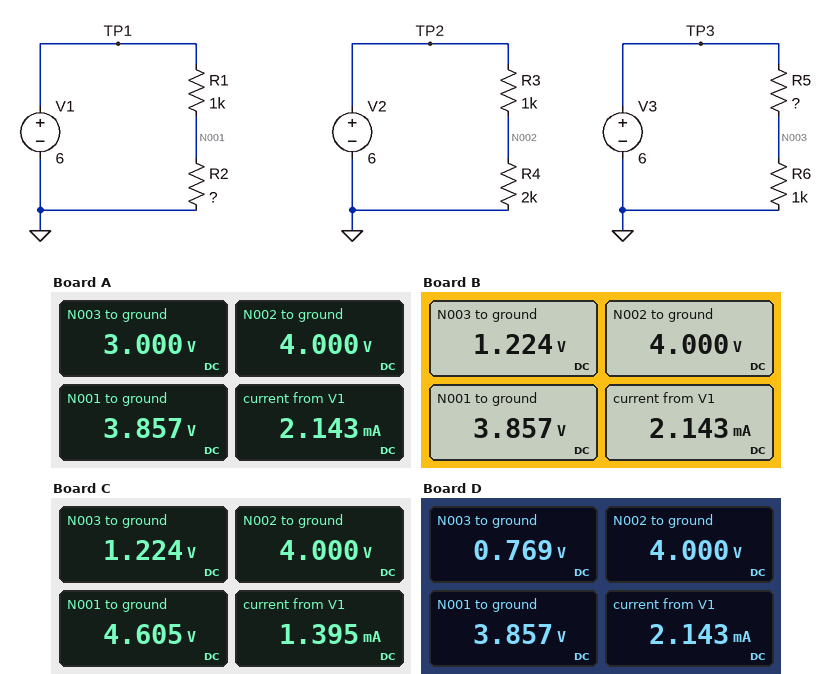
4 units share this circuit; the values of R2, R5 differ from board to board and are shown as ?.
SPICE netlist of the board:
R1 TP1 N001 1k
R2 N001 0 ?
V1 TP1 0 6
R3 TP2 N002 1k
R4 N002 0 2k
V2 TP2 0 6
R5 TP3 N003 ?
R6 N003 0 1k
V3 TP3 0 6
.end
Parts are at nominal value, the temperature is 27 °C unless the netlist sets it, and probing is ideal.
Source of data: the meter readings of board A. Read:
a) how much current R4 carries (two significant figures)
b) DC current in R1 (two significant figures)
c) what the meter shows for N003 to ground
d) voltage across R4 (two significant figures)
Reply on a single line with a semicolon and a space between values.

2.0 mA; 2.1 mA; 3.000 V; 4.0 V
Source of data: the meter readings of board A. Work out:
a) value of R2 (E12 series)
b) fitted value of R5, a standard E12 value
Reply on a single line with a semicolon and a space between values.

1.8 kΩ; 1 kΩ
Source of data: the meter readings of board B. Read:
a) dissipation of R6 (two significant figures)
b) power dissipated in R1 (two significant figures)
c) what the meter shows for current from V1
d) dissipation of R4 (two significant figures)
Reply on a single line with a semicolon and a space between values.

1.5 mW; 4.6 mW; 2.143 mA; 8.0 mW
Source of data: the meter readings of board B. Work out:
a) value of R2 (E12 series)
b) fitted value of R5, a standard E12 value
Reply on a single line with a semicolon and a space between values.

1.8 kΩ; 3.9 kΩ
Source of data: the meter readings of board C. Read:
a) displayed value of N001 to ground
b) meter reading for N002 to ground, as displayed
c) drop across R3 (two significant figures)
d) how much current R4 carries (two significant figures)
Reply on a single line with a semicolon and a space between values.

4.605 V; 4.000 V; 2.0 V; 2.0 mA
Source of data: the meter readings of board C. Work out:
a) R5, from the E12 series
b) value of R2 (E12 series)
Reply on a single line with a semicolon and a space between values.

3.9 kΩ; 3.3 kΩ
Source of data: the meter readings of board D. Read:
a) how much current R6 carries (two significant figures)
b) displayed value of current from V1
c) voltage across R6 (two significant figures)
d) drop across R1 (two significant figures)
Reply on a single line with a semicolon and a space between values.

770 µA; 2.143 mA; 770 mV; 2.1 V
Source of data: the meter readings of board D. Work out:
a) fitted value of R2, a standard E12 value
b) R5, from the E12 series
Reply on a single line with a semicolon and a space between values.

1.8 kΩ; 6.8 kΩ
